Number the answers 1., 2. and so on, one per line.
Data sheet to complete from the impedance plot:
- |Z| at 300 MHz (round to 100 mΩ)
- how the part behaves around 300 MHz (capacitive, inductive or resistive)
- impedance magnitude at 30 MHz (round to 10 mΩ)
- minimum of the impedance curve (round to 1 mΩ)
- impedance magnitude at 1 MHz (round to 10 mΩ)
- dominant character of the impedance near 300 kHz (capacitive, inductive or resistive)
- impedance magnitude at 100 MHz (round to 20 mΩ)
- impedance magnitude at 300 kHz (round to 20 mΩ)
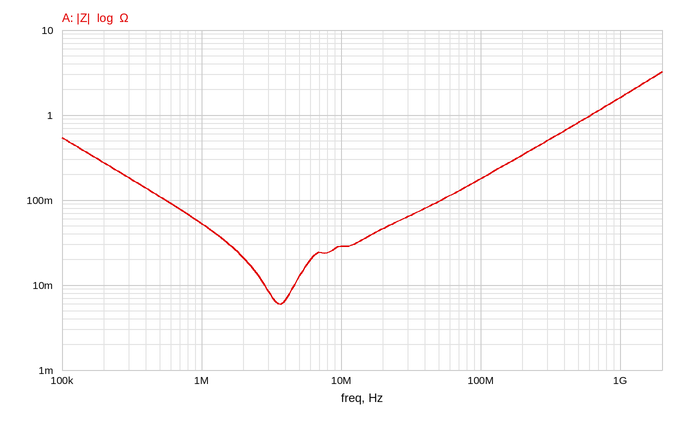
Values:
1. 500 mΩ
2. inductive
3. 60 mΩ
4. 6 mΩ
5. 50 mΩ
6. capacitive
7. 180 mΩ
8. 180 mΩ
